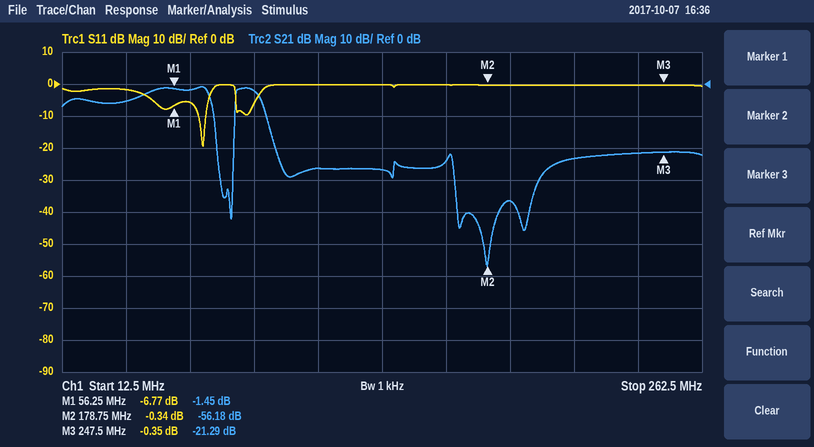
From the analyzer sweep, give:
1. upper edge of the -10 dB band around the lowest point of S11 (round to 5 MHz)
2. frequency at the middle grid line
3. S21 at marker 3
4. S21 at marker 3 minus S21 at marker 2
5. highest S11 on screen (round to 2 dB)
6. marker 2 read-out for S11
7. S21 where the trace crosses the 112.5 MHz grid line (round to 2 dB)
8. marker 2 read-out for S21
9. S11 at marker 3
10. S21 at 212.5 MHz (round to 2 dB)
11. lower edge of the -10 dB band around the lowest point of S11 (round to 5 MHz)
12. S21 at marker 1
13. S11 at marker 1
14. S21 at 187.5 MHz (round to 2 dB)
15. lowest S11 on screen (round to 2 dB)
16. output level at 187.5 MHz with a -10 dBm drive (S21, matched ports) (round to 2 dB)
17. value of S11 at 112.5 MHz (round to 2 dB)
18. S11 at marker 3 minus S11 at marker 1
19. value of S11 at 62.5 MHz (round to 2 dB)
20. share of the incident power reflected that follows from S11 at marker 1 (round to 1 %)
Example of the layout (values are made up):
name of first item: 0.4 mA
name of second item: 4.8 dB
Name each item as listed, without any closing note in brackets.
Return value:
upper edge of the -10 dB band around the lowest point of S11: 70 MHz
frequency at the middle grid line: 137.5 MHz
S21 at marker 3: -21.29 dB
S21 at marker 3 minus S21 at marker 2: 34.89 dB
highest S11 on screen: 0 dB
marker 2 read-out for S11: -0.34 dB
S21 where the trace crosses the 112.5 MHz grid line: -26 dB
marker 2 read-out for S21: -56.18 dB
S11 at marker 3: -0.35 dB
S21 at 212.5 MHz: -24 dB
lower edge of the -10 dB band around the lowest point of S11: 65 MHz
S21 at marker 1: -1.45 dB
S11 at marker 1: -6.77 dB
S21 at 187.5 MHz: -36 dB
lowest S11 on screen: -20 dB
output level at 187.5 MHz with a -10 dBm drive (S21, matched ports): -46 dBm
value of S11 at 112.5 MHz: 0 dB
S11 at marker 3 minus S11 at marker 1: 6.42 dB
value of S11 at 62.5 MHz: -6 dB
share of the incident power reflected that follows from S11 at marker 1: 21 %
